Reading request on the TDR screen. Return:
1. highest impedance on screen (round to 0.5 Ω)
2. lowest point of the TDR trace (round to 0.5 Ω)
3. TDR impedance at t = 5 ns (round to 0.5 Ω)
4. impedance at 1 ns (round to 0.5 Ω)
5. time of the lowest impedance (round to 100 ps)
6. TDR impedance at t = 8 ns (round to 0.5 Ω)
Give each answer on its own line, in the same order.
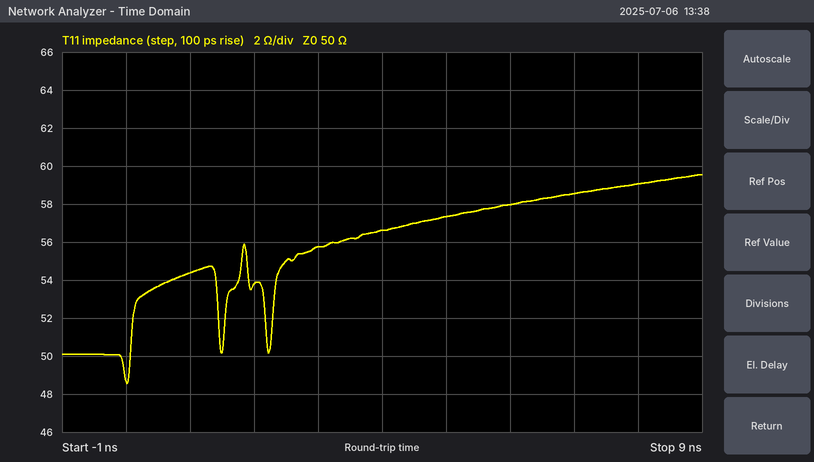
59.5 Ω
48.5 Ω
57.5 Ω
54.5 Ω
0.0 ns
59.0 Ω
